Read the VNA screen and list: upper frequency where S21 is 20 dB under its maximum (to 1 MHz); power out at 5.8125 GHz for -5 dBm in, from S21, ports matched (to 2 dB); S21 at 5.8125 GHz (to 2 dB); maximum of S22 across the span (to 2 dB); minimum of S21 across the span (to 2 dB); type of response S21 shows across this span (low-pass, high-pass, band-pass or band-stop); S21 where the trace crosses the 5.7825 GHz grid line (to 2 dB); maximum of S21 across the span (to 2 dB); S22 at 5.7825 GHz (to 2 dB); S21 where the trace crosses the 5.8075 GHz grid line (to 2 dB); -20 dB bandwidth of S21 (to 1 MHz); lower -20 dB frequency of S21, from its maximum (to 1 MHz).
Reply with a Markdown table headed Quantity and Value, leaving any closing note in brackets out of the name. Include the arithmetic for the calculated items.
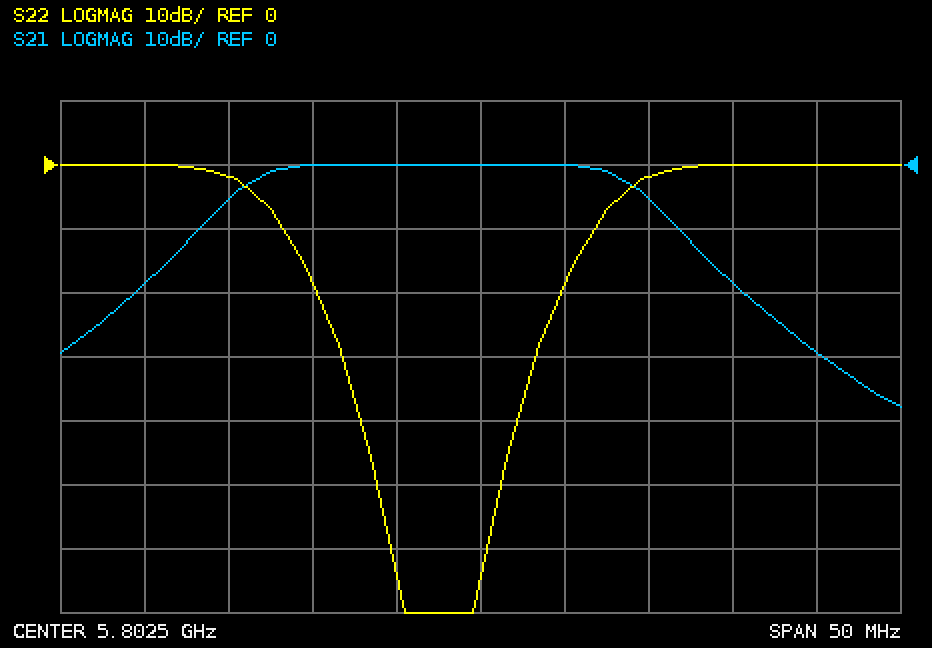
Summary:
| Quantity | Value |
|---|---|
| upper frequency where S21 is 20 dB under its maximum | 5.818 GHz |
| power out at 5.8125 GHz for -5 dBm in, from S21, ports matched | -5 dBm + (-6 dB) = -10 dBm |
| S21 at 5.8125 GHz | -6 dB |
| maximum of S22 across the span | 0 dB |
| minimum of S21 across the span | -38 dB |
| type of response S21 shows across this span | band-pass |
| S21 where the trace crosses the 5.7825 GHz grid line | -18 dB |
| maximum of S21 across the span | 0 dB |
| S22 at 5.7825 GHz | 0 dB |
| S21 where the trace crosses the 5.8075 GHz grid line | 0 dB |
| -20 dB bandwidth of S21 | 5.818 GHz − 5.782 GHz = 36 MHz |
| lower -20 dB frequency of S21, from its maximum | 5.782 GHz |
